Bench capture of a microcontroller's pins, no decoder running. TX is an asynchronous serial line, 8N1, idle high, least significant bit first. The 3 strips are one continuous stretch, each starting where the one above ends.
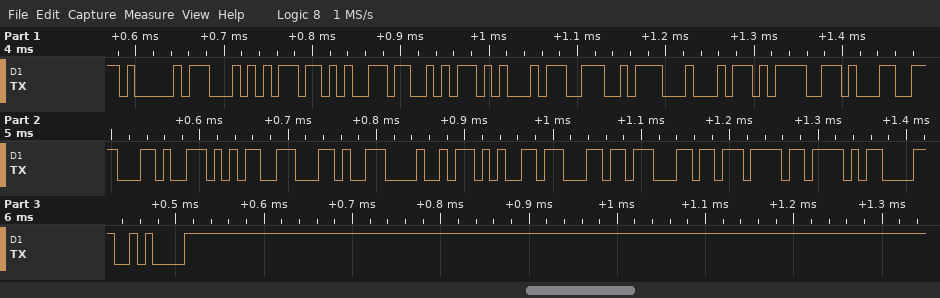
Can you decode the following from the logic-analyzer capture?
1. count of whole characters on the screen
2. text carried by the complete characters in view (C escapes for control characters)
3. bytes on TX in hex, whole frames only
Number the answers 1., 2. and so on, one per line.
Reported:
1. 19
2. "AT+SEND=1,5,Hello\r\n"
3. 41 54 2B 53 45 4E 44 3D 31 2C 35 2C 48 65 6C 6C 6F 0D 0A
